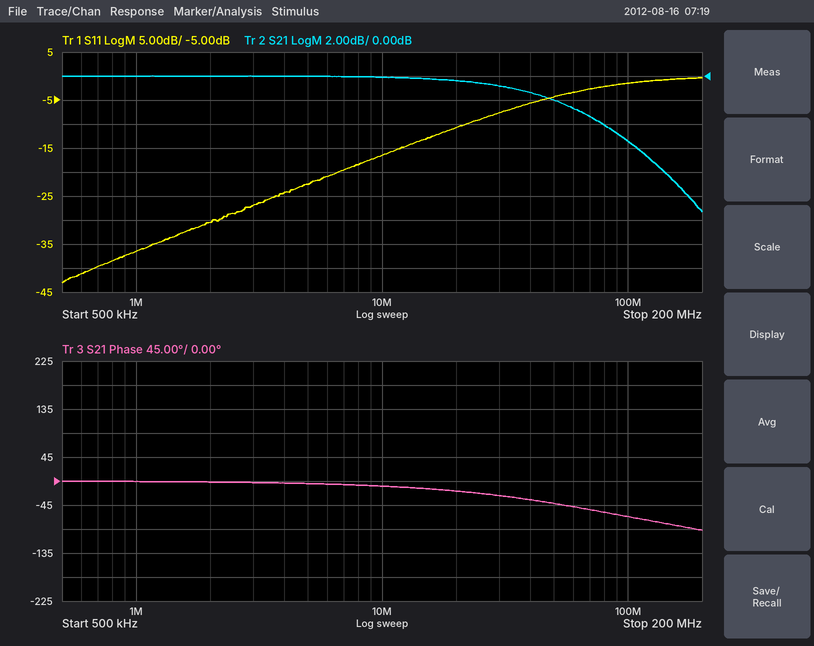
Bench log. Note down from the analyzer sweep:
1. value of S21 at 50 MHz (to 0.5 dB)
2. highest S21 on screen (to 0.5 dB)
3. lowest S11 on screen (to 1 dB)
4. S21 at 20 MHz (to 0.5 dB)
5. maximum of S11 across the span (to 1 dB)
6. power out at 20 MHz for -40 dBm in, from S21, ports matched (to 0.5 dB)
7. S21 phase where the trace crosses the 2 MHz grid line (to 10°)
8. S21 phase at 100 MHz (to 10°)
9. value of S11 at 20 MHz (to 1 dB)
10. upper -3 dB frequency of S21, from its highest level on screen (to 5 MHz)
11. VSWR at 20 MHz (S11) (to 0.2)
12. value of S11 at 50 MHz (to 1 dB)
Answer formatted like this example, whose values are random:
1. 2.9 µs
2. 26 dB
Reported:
1. -2.0 dB
2. 0.0 dB
3. -43 dB
4. -0.5 dB
5. 0 dB
6. -40.5 dBm
7. 0°
8. -70°
9. -11 dB
10. 65 MHz
11. 1.8
12. -4 dB
